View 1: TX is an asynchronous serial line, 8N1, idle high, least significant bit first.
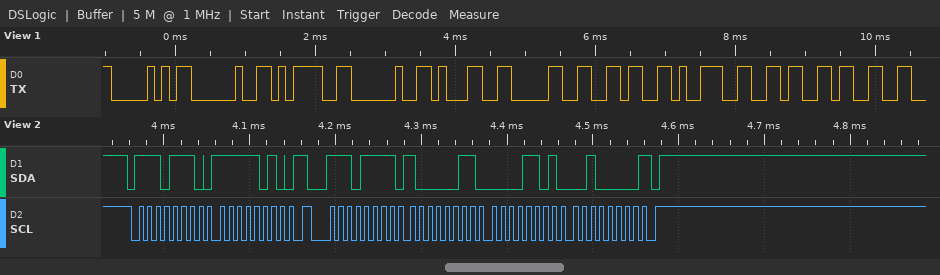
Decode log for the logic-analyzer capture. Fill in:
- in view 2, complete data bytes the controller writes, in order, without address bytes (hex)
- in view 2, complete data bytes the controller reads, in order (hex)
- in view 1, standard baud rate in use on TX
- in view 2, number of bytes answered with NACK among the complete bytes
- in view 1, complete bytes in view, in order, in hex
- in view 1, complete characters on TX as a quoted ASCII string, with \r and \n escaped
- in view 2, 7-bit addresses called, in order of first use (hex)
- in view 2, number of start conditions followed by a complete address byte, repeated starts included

FA
83 0D 20
9600 baud
1
50 20 3D 20 31 30 36 39 36 33
"P = 106963"
0x77
2
